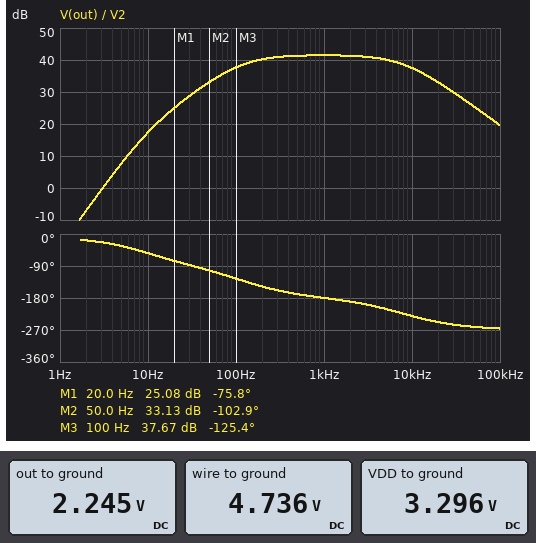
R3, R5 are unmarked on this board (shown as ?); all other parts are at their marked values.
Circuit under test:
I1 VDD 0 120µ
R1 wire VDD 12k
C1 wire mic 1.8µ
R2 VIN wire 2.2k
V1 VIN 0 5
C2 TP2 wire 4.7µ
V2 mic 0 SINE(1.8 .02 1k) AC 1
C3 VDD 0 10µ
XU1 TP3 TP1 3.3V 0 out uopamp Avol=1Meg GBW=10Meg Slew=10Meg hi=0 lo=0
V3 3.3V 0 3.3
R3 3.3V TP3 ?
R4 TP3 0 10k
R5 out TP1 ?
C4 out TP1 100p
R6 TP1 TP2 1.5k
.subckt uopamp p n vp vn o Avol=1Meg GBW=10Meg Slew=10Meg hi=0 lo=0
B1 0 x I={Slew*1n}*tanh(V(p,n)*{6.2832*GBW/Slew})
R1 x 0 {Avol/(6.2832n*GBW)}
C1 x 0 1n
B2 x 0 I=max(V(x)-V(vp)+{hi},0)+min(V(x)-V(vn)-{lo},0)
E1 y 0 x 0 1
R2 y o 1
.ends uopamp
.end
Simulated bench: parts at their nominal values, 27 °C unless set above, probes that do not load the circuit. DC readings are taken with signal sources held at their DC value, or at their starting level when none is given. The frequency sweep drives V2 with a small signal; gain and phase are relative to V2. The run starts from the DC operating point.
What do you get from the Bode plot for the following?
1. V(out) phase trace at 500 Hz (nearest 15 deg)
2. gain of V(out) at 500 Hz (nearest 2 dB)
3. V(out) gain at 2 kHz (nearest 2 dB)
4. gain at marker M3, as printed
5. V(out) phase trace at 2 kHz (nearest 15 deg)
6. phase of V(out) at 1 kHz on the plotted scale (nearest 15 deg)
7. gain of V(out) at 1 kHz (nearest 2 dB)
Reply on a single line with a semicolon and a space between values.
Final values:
-165 deg; 42 dB; 42 dB; 37.67 dB; -195 deg; -180 deg; 42 dB
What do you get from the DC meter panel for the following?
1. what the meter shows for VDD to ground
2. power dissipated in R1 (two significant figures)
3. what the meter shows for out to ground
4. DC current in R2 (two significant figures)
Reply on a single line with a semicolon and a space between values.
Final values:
3.296 V; 170 µW; 2.245 V; 120 µA
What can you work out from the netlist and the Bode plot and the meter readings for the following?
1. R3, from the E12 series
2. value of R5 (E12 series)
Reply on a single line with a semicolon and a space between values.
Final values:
4.7 kΩ; 180 kΩ
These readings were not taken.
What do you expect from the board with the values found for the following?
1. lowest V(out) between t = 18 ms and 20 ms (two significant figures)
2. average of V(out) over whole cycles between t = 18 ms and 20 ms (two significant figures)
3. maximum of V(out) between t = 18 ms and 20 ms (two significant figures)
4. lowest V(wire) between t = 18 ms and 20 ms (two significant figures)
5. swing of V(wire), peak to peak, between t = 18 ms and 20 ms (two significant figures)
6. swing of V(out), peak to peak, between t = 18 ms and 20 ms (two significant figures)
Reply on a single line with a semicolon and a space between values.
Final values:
260 mV; 2.2 V; 3.3 V; 4.7 V; 40 mV; 3.0 V
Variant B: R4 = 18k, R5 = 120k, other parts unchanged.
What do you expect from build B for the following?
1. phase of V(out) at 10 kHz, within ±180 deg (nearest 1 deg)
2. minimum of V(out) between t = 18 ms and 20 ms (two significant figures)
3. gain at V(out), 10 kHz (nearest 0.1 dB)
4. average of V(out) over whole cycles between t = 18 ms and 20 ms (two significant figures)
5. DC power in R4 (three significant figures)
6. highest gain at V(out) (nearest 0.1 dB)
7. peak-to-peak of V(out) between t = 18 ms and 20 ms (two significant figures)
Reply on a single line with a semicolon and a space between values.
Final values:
141 deg; 1.3 V; 35.8 dB; 2.6 V; 380 µW; 38.0 dB; 2.0 V
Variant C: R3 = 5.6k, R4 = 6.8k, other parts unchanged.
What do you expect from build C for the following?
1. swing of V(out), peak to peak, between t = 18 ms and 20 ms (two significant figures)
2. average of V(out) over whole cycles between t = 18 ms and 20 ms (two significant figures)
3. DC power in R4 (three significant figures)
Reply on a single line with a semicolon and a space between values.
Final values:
3.3 V; 1.8 V; 482 µW
